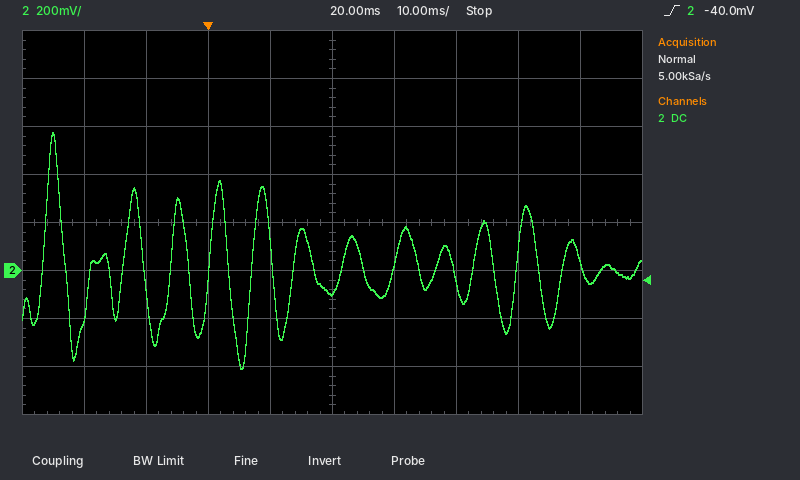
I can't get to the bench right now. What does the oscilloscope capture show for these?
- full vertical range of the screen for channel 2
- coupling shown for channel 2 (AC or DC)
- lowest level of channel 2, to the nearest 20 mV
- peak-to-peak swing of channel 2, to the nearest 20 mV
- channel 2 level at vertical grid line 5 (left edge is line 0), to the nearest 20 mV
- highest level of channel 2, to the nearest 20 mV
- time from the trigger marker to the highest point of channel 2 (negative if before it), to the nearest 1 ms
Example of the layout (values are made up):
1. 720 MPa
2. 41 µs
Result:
1. 1.6 V
2. DC
3. -400 mV
4. 980 mV
5. -100 mV
6. 580 mV
7. -25 ms
